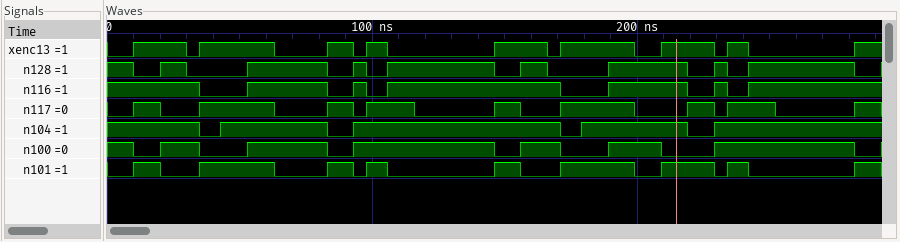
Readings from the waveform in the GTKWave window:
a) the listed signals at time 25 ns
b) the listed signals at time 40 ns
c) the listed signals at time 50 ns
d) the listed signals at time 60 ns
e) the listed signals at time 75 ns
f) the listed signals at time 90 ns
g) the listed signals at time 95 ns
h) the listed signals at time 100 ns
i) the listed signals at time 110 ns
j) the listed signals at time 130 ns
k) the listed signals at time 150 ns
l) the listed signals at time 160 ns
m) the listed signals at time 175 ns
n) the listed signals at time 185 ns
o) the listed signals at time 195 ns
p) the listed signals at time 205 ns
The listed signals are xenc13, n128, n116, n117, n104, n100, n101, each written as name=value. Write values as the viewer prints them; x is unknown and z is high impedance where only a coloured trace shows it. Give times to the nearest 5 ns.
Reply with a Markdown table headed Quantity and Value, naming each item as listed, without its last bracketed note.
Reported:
| Quantity | Value |
|---|---|
| the listed signals at time 25 ns | xenc13=1, n128=1, n116=1, n117=0, n104=1, n100=1, n101=0 |
| the listed signals at time 40 ns | xenc13=1, n128=0, n116=0, n117=1, n104=0, n100=0, n101=1 |
| the listed signals at time 50 ns | xenc13=1, n128=0, n116=0, n117=1, n104=1, n100=0, n101=1 |
| the listed signals at time 60 ns | xenc13=1, n128=1, n116=1, n117=1, n104=1, n100=1, n101=1 |
| the listed signals at time 75 ns | xenc13=0, n128=1, n116=1, n117=0, n104=1, n100=1, n101=0 |
| the listed signals at time 90 ns | xenc13=1, n128=0, n116=0, n117=1, n104=0, n100=0, n101=1 |
| the listed signals at time 95 ns | xenc13=0, n128=1, n116=1, n117=0, n104=1, n100=1, n101=0 |
| the listed signals at time 100 ns | xenc13=1, n128=0, n116=0, n117=1, n104=1, n100=1, n101=1 |
| the listed signals at time 110 ns | xenc13=0, n128=1, n116=1, n117=1, n104=1, n100=1, n101=0 |
| the listed signals at time 130 ns | xenc13=0, n128=1, n116=1, n117=0, n104=1, n100=1, n101=0 |
| the listed signals at time 150 ns | xenc13=1, n128=0, n116=1, n117=1, n104=1, n100=0, n101=1 |
| the listed signals at time 160 ns | xenc13=1, n128=1, n116=1, n117=0, n104=1, n100=1, n101=0 |
| the listed signals at time 175 ns | xenc13=1, n128=0, n116=0, n117=1, n104=0, n100=0, n101=1 |
| the listed signals at time 185 ns | xenc13=1, n128=0, n116=0, n117=1, n104=1, n100=0, n101=1 |
| the listed signals at time 195 ns | xenc13=1, n128=1, n116=1, n117=1, n104=1, n100=1, n101=1 |
| the listed signals at time 205 ns | xenc13=0, n128=1, n116=1, n117=0, n104=1, n100=1, n101=0 |
